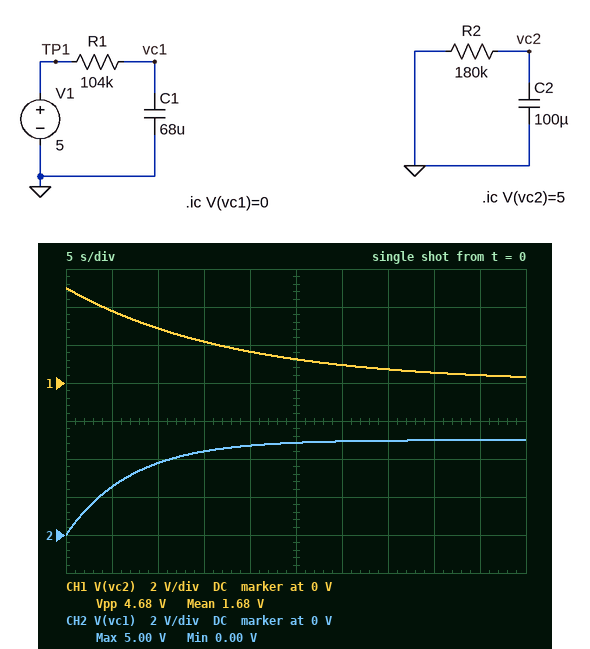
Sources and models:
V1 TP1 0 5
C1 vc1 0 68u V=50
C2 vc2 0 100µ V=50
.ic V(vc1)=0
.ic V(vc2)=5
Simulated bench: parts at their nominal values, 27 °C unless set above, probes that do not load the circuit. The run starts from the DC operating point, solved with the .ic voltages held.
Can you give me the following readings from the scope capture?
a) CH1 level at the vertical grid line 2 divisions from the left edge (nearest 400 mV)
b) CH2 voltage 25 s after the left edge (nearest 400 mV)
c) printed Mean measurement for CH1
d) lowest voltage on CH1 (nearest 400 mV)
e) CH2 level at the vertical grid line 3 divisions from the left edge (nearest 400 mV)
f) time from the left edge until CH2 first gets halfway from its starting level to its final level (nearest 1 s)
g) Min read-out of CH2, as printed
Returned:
2.8 V
4.8 V
1.68 V
400 mV
4.4 V
5 s
0.00 V
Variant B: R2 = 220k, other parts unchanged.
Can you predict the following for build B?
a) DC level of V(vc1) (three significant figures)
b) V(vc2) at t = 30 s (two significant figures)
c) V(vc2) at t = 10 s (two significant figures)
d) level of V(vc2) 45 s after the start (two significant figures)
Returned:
5.00 V
1.3 V
3.2 V
650 mV
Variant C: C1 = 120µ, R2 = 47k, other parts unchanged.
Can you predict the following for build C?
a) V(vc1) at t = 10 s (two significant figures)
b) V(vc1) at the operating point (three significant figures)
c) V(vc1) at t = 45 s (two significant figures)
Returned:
2.8 V
5.00 V
4.9 V
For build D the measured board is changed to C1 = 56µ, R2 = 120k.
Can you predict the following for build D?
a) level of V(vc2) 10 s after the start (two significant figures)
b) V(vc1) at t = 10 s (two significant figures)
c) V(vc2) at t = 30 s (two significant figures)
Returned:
2.2 V
4.1 V
410 mV
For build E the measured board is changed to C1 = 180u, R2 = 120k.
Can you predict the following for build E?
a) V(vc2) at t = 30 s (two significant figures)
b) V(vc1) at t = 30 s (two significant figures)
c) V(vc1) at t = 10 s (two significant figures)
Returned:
410 mV
4.0 V
2.1 V
